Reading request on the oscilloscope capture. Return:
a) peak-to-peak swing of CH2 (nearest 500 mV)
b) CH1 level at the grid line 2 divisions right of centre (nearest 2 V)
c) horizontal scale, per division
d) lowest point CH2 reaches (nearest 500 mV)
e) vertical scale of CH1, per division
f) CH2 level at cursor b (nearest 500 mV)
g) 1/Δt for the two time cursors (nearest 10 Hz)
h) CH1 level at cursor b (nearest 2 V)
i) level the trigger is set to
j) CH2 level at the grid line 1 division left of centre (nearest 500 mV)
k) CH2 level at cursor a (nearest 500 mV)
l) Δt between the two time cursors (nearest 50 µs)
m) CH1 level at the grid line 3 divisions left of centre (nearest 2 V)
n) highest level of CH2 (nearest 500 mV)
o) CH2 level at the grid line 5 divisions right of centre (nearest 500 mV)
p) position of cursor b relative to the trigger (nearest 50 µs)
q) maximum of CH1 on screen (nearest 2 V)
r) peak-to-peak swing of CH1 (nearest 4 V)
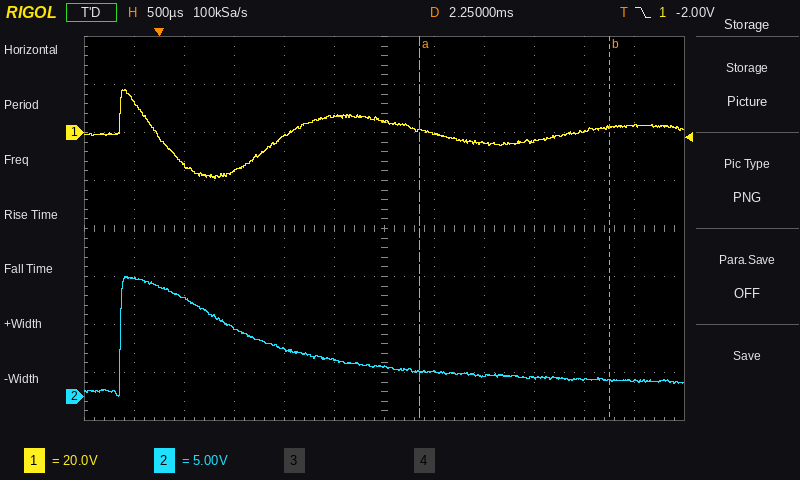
12.5 V
-4 V
500 µs
0.0 V
20 V
1.5 V
530 Hz
2 V
-2.00 V
4.0 V
2.5 V
1.90 ms
-16 V
12.5 V
1.5 V
+4.50 ms
18 V
36 V
